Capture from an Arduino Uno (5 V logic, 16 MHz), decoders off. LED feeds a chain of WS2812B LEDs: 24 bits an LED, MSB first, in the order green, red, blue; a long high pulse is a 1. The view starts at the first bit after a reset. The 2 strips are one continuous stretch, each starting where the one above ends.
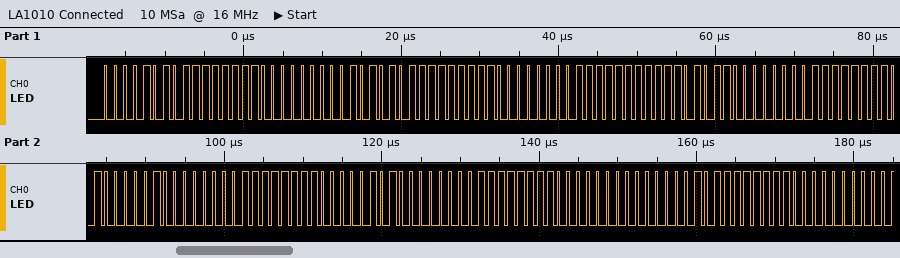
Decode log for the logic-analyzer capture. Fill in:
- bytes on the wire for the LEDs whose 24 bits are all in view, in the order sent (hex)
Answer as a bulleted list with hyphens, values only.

- 0A FF 00 55 FF 00 FF EB 00 FF 41 00 FF 05 00 FF 00 02
